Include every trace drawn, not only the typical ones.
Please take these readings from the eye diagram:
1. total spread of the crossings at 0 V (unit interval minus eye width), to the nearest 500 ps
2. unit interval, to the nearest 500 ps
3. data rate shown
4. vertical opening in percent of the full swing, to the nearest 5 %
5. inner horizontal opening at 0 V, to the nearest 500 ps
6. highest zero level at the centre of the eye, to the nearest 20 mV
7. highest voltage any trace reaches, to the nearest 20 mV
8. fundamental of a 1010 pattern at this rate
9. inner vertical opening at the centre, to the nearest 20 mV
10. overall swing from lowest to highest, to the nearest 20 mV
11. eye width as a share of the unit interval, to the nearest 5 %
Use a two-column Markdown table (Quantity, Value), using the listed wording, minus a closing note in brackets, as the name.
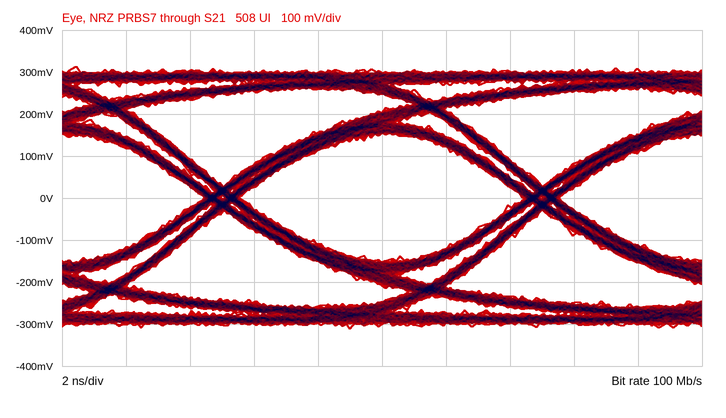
| Quantity | Value |
|---|---|
| total spread of the crossings at 0 V (unit interval minus eye width), to the nearest 500 ps | 1.0 ns |
| unit interval, to the nearest 500 ps | 10.0 ns |
| data rate shown | 100 Mb/s |
| vertical opening in percent of the full swing, to the nearest 5 % | 50 % |
| inner horizontal opening at 0 V, to the nearest 500 ps | 9.0 ns |
| highest zero level at the centre of the eye, to the nearest 20 mV | -160 mV |
| highest voltage any trace reaches, to the nearest 20 mV | 320 mV |
| fundamental of a 1010 pattern at this rate | 50 MHz |
| inner vertical opening at the centre, to the nearest 20 mV | 300 mV |
| overall swing from lowest to highest, to the nearest 20 mV | 620 mV |
| eye width as a share of the unit interval, to the nearest 5 % | 90 % |
